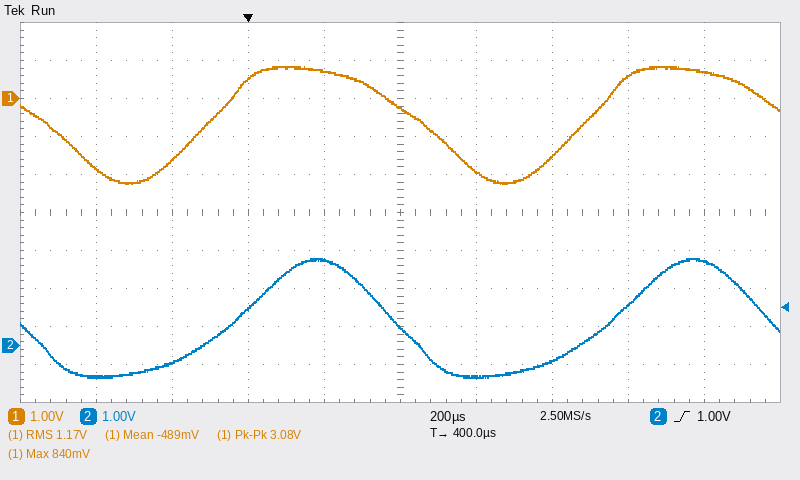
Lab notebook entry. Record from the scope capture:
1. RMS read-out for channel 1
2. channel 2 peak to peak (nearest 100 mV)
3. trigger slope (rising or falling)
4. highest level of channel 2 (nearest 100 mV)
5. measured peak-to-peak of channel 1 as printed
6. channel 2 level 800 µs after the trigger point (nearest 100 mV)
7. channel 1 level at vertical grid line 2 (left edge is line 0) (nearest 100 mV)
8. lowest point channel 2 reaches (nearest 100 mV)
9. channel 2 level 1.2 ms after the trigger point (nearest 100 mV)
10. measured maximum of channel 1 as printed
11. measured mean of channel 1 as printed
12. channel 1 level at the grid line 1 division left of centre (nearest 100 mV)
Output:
1.17 V
3.1 V
rising
2.3 V
3.08 V
-400 mV
-1.6 V
-800 mV
2.2 V
840 mV
-489 mV
700 mV
